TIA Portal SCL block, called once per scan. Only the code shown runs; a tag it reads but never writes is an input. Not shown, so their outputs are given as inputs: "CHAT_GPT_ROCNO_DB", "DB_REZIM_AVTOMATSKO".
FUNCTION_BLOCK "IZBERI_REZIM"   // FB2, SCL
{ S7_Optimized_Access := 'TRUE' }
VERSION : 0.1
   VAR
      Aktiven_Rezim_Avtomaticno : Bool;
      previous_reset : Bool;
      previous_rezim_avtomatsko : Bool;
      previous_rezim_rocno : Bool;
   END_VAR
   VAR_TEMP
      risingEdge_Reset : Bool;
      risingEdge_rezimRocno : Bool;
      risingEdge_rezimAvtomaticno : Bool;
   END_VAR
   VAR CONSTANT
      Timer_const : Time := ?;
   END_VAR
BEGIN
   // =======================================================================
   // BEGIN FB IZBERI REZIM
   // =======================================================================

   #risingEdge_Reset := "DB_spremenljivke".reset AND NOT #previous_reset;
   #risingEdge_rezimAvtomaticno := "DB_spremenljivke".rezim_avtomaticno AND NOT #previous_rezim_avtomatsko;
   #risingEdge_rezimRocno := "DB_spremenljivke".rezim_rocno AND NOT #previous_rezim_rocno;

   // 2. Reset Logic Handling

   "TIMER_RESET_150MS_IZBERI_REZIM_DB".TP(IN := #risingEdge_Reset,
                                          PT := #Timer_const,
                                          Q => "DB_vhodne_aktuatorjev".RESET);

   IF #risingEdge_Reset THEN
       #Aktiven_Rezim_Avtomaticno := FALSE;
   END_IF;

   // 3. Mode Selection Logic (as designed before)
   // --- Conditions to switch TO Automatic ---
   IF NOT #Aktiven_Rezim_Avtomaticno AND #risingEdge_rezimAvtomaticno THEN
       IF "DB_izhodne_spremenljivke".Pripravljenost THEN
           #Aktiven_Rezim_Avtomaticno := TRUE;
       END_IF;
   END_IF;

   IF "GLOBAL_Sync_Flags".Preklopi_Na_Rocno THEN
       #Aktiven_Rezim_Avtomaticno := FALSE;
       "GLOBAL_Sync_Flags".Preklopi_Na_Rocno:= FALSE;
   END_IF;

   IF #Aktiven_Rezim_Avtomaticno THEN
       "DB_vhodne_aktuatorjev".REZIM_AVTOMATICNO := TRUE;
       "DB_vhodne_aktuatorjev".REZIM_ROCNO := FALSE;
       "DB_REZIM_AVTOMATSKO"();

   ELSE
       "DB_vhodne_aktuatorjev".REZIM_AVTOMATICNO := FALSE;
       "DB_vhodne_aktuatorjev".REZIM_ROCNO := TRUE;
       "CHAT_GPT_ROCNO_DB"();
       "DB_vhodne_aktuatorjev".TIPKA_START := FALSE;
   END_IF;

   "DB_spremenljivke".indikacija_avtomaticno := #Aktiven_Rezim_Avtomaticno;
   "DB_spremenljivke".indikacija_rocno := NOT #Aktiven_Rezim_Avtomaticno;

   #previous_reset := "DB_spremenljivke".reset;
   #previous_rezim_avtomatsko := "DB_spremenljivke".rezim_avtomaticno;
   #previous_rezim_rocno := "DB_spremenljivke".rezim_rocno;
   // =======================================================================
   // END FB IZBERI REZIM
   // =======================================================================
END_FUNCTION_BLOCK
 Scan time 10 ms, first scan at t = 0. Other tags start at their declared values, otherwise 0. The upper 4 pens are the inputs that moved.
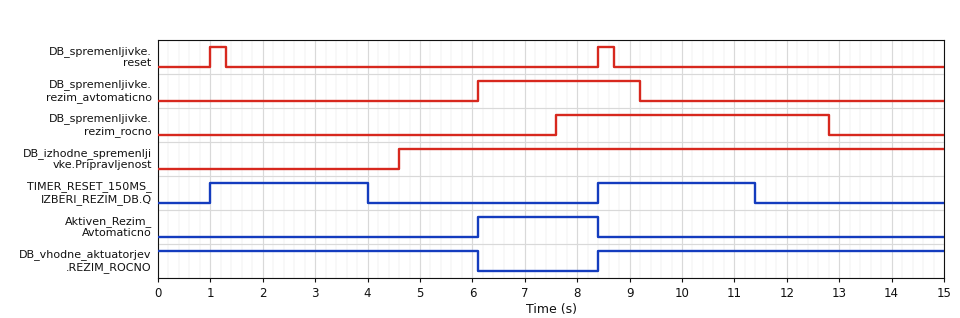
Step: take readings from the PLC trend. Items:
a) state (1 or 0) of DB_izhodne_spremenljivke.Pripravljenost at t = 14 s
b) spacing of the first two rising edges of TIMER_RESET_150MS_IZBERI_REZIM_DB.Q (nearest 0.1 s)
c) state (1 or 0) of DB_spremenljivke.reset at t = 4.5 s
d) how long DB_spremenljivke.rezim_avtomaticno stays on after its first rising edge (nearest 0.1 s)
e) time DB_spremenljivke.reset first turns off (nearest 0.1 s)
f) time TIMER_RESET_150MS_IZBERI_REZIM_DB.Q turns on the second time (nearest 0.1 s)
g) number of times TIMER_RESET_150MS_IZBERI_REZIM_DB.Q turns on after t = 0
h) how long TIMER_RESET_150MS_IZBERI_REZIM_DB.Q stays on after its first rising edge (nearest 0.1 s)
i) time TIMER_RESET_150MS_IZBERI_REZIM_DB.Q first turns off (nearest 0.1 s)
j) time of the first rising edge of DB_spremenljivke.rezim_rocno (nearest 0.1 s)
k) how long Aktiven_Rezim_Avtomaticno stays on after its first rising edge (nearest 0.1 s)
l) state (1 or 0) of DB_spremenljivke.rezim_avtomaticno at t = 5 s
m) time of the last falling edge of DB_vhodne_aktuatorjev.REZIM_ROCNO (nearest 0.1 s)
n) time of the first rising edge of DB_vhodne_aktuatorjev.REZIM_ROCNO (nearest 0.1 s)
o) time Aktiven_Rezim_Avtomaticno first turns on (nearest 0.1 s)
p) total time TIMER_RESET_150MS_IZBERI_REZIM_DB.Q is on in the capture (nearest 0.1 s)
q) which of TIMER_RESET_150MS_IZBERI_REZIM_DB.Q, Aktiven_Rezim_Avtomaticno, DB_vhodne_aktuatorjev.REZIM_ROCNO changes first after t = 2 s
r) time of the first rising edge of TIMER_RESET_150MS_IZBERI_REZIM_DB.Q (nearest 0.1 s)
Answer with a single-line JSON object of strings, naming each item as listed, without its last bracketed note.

{"state (1 or 0) of DB_izhodne_spremenljivke.Pripravljenost at t = 14 s": "1", "spacing of the first two rising edges of TIMER_RESET_150MS_IZBERI_REZIM_DB.Q": "7.4 s", "state (1 or 0) of DB_spremenljivke.reset at t = 4.5 s": "0", "how long DB_spremenljivke.rezim_avtomaticno stays on after its first rising edge": "3.1 s", "time DB_spremenljivke.reset first turns off": "1.3 s", "time TIMER_RESET_150MS_IZBERI_REZIM_DB.Q turns on the second time": "8.4 s", "number of times TIMER_RESET_150MS_IZBERI_REZIM_DB.Q turns on after t = 0": "2", "how long TIMER_RESET_150MS_IZBERI_REZIM_DB.Q stays on after its first rising edge": "3.0 s", "time TIMER_RESET_150MS_IZBERI_REZIM_DB.Q first turns off": "4.0 s", "time of the first rising edge of DB_spremenljivke.rezim_rocno": "7.6 s", "how long Aktiven_Rezim_Avtomaticno stays on after its first rising edge": "2.3 s", "state (1 or 0) of DB_spremenljivke.rezim_avtomaticno at t = 5 s": "0", "time of the last falling edge of DB_vhodne_aktuatorjev.REZIM_ROCNO": "6.1 s", "time of the first rising edge of DB_vhodne_aktuatorjev.REZIM_ROCNO": "8.4 s", "time Aktiven_Rezim_Avtomaticno first turns on": "6.1 s", "total time TIMER_RESET_150MS_IZBERI_REZIM_DB.Q is on in the capture": "6.0 s", "which of TIMER_RESET_150MS_IZBERI_REZIM_DB.Q, Aktiven_Rezim_Avtomaticno, DB_vhodne_aktuatorjev.REZIM_ROCNO changes first after t = 2 s": "TIMER_RESET_150MS_IZBERI_REZIM_DB.Q", "time of the first rising edge of TIMER_RESET_150MS_IZBERI_REZIM_DB.Q": "1.0 s"}
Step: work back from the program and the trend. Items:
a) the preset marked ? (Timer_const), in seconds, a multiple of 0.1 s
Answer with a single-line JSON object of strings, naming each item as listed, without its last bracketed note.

{"the preset marked ? (Timer_const), in seconds, a multiple of 0.1 s": "3.0 s"}
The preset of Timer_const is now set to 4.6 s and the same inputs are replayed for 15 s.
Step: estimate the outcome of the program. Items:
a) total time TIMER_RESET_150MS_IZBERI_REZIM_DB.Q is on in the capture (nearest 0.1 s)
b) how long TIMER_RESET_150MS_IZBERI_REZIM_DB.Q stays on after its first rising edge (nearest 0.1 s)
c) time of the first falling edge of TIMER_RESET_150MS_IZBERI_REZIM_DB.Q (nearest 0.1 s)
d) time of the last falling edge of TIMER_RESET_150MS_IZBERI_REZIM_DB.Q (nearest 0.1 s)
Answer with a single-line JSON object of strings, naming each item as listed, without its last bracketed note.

{"total time TIMER_RESET_150MS_IZBERI_REZIM_DB.Q is on in the capture": "9.2 s", "how long TIMER_RESET_150MS_IZBERI_REZIM_DB.Q stays on after its first rising edge": "4.6 s", "time of the first falling edge of TIMER_RESET_150MS_IZBERI_REZIM_DB.Q": "5.6 s", "time of the last falling edge of TIMER_RESET_150MS_IZBERI_REZIM_DB.Q": "13.0 s"}
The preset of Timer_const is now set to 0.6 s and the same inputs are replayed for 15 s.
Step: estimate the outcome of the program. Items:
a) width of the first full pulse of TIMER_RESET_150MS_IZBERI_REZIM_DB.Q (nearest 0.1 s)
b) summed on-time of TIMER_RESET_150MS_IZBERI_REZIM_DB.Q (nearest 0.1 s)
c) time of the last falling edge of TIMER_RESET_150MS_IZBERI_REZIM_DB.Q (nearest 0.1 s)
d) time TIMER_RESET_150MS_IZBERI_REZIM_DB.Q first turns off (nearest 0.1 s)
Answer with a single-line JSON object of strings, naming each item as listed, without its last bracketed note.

{"width of the first full pulse of TIMER_RESET_150MS_IZBERI_REZIM_DB.Q": "0.6 s", "summed on-time of TIMER_RESET_150MS_IZBERI_REZIM_DB.Q": "1.2 s", "time of the last falling edge of TIMER_RESET_150MS_IZBERI_REZIM_DB.Q": "9.0 s", "time TIMER_RESET_150MS_IZBERI_REZIM_DB.Q first turns off": "1.6 s"}
